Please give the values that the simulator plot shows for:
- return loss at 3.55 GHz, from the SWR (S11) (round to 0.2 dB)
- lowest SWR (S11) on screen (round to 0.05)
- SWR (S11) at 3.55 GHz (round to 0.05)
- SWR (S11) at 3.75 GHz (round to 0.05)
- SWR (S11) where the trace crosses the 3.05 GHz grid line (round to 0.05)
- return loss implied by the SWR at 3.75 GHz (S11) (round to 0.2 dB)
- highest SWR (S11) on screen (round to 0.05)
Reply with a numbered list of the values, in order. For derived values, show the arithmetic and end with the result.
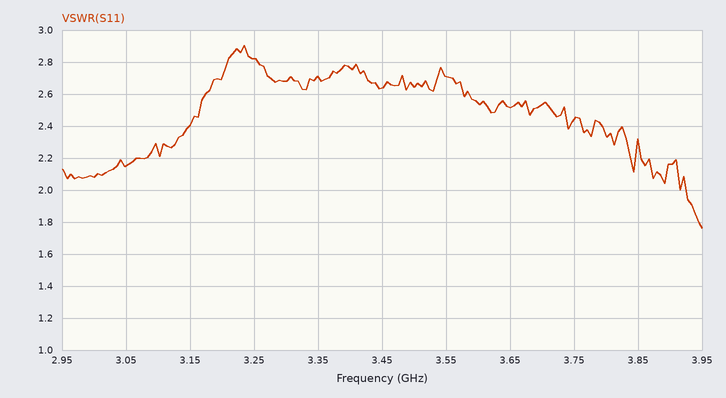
1. −20 log10((2.7 − 1)/(2.7 + 1)) ≈ 6.8 dB
2. 1.75
3. 2.70
4. 2.45
5. 2.15
6. −20 log10((2.45 − 1)/(2.45 + 1)) ≈ 7.53 dB, so 7.6 dB to the nearest 0.2 dB
7. 2.90
